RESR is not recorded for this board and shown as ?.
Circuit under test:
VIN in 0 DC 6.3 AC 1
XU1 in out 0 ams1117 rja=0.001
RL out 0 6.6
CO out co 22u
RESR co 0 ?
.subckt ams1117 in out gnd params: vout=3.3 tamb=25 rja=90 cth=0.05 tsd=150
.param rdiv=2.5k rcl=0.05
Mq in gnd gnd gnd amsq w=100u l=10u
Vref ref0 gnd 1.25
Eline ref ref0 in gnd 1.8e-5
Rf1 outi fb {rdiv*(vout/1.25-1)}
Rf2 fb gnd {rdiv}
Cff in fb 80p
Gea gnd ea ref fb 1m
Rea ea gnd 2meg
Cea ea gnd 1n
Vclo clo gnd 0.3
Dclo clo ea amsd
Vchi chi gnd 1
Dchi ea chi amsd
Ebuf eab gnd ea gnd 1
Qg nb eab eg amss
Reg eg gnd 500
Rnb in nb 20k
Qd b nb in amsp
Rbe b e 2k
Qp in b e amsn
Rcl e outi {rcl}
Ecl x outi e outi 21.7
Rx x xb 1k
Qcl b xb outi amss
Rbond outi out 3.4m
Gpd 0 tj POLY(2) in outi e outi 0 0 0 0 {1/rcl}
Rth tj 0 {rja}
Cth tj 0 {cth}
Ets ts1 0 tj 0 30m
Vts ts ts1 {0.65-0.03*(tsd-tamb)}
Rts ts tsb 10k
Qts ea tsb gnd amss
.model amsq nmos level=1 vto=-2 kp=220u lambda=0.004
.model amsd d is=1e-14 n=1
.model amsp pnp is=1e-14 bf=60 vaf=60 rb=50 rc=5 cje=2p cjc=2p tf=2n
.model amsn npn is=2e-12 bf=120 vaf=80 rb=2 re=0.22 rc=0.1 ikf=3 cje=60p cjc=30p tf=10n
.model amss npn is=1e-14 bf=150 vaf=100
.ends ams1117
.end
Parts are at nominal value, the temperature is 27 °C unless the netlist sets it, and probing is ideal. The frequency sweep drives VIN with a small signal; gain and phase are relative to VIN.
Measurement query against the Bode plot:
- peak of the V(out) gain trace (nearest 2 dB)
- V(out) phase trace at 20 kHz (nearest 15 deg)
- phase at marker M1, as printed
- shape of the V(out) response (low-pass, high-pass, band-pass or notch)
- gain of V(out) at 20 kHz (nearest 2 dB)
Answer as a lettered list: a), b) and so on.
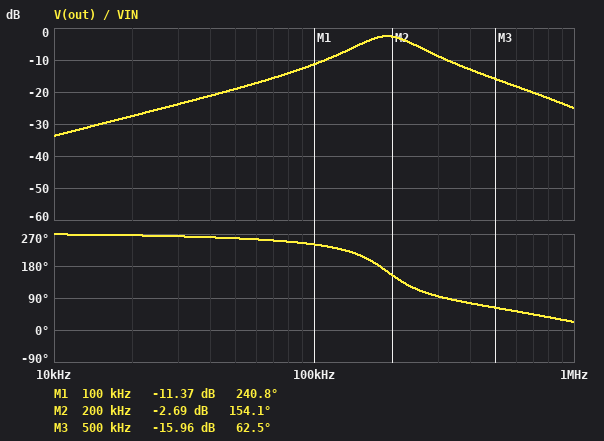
a) -2 dB
b) 270 deg
c) 240.8 deg
d) band-pass
e) -28 dB
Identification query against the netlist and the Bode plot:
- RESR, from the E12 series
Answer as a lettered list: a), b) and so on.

a) 0.56 Ω
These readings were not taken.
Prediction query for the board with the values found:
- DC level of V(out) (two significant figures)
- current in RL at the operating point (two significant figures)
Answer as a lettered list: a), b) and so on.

a) 3.3 V
b) 500 mA
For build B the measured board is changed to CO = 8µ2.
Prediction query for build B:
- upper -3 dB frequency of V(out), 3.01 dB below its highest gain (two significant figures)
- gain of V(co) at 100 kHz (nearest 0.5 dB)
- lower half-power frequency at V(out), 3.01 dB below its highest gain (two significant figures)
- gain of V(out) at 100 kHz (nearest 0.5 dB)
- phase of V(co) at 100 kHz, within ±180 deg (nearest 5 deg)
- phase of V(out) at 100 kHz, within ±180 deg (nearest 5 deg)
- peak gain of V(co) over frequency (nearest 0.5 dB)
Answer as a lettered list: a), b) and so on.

a) 230 kHz
b) -11.0 dB
c) 150 kHz
d) -10.5 dB
e) -95 deg
f) -115 deg
g) -0.5 dB
